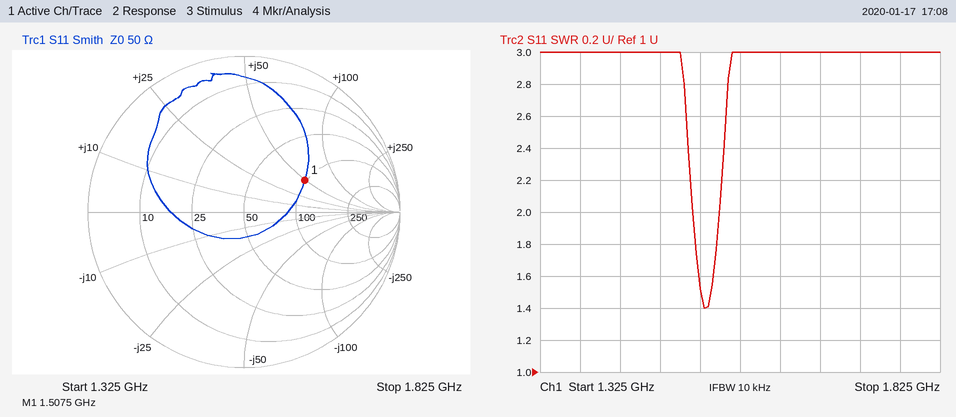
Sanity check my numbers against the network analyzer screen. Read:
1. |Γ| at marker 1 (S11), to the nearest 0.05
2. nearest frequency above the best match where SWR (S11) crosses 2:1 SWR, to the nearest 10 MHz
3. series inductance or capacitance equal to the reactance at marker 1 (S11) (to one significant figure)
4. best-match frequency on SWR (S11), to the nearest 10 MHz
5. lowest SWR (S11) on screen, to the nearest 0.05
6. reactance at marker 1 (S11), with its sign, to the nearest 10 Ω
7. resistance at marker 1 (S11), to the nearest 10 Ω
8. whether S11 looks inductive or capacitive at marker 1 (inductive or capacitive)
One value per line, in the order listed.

0.45
1.55 GHz
5 nH
1.53 GHz
1.40
+50 Ω
100 Ω
inductive
